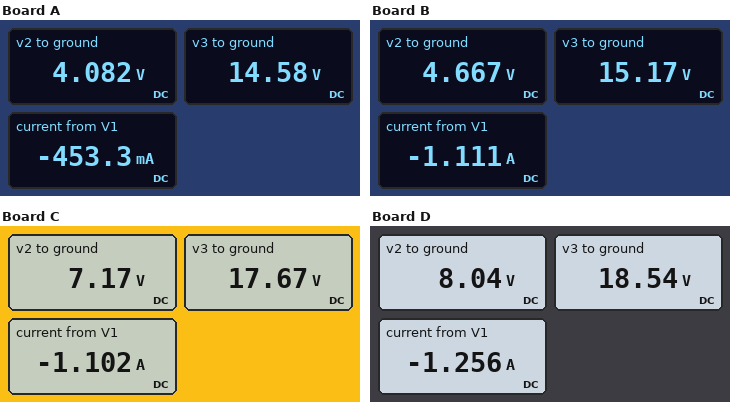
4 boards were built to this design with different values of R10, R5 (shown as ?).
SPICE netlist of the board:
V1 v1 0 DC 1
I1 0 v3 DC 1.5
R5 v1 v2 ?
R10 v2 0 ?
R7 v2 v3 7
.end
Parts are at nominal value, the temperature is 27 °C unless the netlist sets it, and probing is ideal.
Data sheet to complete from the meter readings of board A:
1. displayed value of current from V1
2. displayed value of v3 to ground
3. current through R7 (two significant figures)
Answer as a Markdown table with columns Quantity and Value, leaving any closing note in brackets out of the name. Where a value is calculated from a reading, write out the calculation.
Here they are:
| Quantity | Value |
|---|---|
| displayed value of current from V1 | -453.3 mA |
| displayed value of v3 to ground | 14.58 V |
| current through R7 | (14.58 V - 4.082 V) / 7 Ω = 1.5 A |
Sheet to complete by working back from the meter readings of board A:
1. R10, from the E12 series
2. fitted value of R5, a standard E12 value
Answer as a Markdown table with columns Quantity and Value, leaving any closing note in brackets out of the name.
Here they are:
| Quantity | Value |
|---|---|
| R10, from the E12 series | 3.9 Ω |
| fitted value of R5, a standard E12 value | 6.8 Ω |
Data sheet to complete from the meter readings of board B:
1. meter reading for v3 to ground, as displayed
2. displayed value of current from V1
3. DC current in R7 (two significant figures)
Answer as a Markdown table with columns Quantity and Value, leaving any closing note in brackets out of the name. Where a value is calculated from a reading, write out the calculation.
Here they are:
| Quantity | Value |
|---|---|
| meter reading for v3 to ground, as displayed | 15.17 V |
| displayed value of current from V1 | -1.111 A |
| DC current in R7 | (15.17 V - 4.667 V) / 7 Ω = 1.5 A |
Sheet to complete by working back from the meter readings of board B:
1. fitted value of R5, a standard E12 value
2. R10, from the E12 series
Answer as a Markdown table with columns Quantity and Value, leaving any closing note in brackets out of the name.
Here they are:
| Quantity | Value |
|---|---|
| fitted value of R5, a standard E12 value | 3.3 Ω |
| R10, from the E12 series | 12 Ω |
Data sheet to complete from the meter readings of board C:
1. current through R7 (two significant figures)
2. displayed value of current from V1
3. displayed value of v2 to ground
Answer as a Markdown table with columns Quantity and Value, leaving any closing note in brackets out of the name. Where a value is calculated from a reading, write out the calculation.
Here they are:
| Quantity | Value |
|---|---|
| current through R7 | (17.67 V - 7.17 V) / 7 Ω = 1.5 A |
| displayed value of current from V1 | -1.102 A |
| displayed value of v2 to ground | 7.17 V |
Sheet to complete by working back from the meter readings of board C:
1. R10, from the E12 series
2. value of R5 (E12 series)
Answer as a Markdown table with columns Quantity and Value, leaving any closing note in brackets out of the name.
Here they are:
| Quantity | Value |
|---|---|
| R10, from the E12 series | 18 Ω |
| value of R5 | 5.6 Ω |
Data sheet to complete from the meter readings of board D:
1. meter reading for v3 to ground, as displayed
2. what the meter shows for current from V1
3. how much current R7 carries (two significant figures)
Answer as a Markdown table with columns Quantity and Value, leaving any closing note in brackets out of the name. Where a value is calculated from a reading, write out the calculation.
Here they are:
| Quantity | Value |
|---|---|
| meter reading for v3 to ground, as displayed | 18.54 V |
| what the meter shows for current from V1 | -1.256 A |
| how much current R7 carries | (18.54 V - 8.04 V) / 7 Ω = 1.5 A |
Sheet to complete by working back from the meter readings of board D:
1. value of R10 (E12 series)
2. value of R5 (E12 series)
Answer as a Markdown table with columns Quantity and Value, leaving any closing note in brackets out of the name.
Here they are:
| Quantity | Value |
|---|---|
| value of R10 | 33 Ω |
| value of R5 | 5.6 Ω |
